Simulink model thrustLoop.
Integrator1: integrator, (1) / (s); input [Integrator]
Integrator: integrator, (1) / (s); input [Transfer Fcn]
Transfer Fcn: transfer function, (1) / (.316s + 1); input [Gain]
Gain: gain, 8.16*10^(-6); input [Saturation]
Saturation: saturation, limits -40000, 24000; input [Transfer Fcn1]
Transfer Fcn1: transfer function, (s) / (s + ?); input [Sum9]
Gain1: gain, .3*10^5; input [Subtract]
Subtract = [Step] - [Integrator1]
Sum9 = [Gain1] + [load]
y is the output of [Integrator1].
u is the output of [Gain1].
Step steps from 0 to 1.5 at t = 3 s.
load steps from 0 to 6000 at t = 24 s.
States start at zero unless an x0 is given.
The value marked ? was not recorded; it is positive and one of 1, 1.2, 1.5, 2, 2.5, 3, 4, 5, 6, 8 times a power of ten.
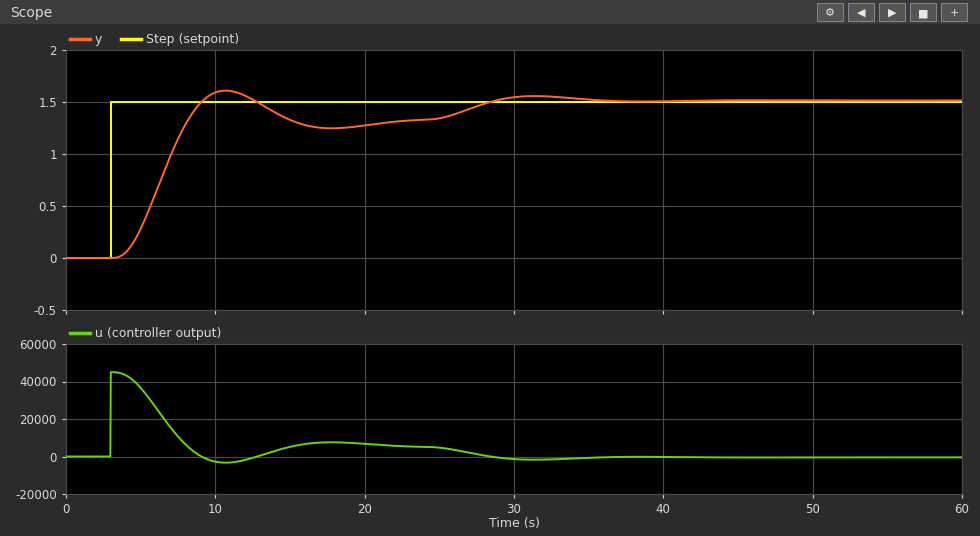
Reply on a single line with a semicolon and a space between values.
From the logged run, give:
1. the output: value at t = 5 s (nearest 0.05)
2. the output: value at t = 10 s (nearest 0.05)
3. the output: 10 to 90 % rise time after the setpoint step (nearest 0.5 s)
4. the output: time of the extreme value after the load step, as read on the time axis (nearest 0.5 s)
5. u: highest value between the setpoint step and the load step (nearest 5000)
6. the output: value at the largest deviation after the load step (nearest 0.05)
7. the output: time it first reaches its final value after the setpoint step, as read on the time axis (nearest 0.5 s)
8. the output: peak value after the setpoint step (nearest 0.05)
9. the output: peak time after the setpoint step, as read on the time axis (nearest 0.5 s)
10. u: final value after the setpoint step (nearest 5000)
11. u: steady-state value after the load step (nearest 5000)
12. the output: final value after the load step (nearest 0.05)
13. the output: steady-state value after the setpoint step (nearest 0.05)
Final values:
0.30; 1.60; 3.0 s; 31.5 s; 45000; 1.55; 8.0 s; 1.60; 10.5 s; 5000; 0; 1.50; 1.30
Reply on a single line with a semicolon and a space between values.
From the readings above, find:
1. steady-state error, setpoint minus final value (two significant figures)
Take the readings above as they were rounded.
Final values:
0.20
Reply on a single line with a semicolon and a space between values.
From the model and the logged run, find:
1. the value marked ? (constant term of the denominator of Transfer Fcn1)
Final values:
0.5
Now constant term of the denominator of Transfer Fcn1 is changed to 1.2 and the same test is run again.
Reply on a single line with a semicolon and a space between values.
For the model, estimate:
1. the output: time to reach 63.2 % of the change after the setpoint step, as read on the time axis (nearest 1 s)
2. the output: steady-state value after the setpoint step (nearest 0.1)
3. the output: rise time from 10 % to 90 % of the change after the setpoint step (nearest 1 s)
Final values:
8 s; 1.3; 8 s
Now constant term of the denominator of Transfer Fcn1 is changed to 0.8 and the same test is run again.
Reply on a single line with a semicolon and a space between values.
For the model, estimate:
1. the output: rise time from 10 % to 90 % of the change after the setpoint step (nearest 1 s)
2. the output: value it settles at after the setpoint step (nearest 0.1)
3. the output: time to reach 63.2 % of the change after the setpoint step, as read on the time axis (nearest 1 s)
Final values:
5 s; 1.3; 7 s
